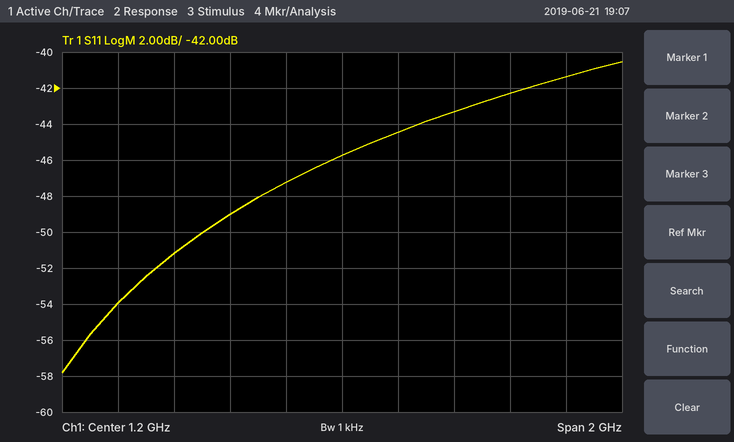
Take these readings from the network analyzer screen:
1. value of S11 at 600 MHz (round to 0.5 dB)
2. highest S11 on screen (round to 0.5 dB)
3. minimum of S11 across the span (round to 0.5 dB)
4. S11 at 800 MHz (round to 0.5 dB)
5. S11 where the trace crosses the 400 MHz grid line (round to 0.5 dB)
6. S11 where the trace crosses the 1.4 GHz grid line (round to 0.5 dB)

-51.0 dB
-40.5 dB
-58.0 dB
-49.0 dB
-54.0 dB
-44.5 dB
